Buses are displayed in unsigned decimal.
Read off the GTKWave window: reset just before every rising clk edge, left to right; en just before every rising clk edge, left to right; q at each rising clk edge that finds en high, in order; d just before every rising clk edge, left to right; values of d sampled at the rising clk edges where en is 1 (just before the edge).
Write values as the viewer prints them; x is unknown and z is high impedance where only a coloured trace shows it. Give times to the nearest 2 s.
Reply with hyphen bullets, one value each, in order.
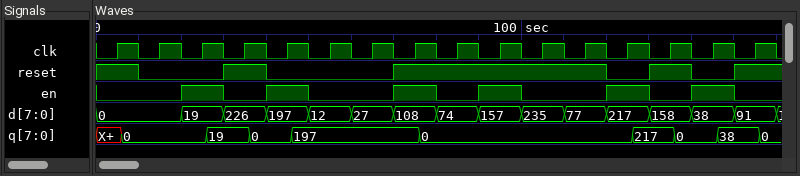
- 1 0 0 1 0 0 0 1 1 1 1 1 0 1 0 1
- 0 0 1 0 1 0 0 1 0 1 0 0 1 0 1 0
- 0, 0, 197, 0, 0, 0
- 0, 0, 19, 226, 197, 12, 27, 108, 74, 157, 235, 77, 217, 158, 38, 91
- 19, 197, 108, 157, 217, 38
